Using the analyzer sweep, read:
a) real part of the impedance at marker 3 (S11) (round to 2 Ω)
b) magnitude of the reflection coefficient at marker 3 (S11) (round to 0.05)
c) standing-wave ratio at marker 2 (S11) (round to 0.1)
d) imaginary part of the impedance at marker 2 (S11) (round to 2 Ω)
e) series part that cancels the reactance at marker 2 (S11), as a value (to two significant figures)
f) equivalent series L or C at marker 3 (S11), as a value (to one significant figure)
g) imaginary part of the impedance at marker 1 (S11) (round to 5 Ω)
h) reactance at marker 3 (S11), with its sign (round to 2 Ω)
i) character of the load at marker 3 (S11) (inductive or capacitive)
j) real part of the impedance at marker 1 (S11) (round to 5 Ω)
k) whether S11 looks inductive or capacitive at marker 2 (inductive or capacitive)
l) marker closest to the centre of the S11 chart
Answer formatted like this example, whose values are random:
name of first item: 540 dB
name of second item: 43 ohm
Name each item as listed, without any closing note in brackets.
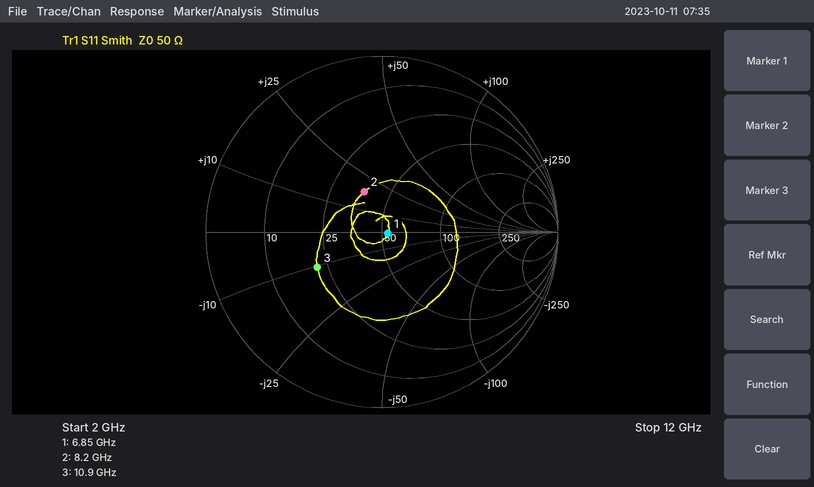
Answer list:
real part of the impedance at marker 3 (S11): 22 Ω
magnitude of the reflection coefficient at marker 3 (S11): 0.40
standing-wave ratio at marker 2 (S11): 1.7
imaginary part of the impedance at marker 2 (S11): +18 Ω
series part that cancels the reactance at marker 2 (S11), as a value: 1.1 pF
equivalent series L or C at marker 3 (S11), as a value: 1 pF
imaginary part of the impedance at marker 1 (S11): 0 Ω
reactance at marker 3 (S11), with its sign: -10 Ω
character of the load at marker 3 (S11): capacitive
real part of the impedance at marker 1 (S11): 55 Ω
whether S11 looks inductive or capacitive at marker 2: inductive
marker closest to the centre of the S11 chart: marker 1
